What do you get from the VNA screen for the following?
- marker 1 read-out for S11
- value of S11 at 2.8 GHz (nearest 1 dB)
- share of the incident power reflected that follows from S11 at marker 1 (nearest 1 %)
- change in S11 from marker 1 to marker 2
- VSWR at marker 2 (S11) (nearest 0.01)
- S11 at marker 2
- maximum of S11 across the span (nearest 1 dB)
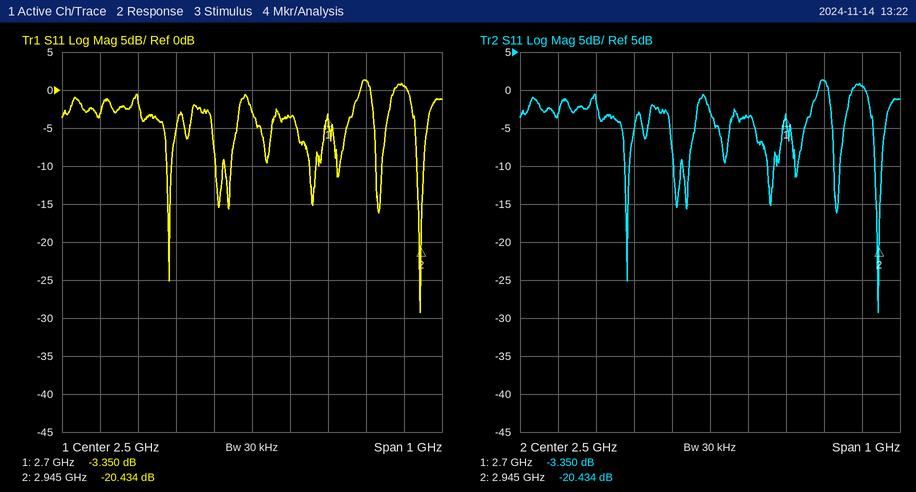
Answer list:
-3.350 dB
1 dB
46 %
-17.084 dB
1.21
-20.434 dB
1 dB
